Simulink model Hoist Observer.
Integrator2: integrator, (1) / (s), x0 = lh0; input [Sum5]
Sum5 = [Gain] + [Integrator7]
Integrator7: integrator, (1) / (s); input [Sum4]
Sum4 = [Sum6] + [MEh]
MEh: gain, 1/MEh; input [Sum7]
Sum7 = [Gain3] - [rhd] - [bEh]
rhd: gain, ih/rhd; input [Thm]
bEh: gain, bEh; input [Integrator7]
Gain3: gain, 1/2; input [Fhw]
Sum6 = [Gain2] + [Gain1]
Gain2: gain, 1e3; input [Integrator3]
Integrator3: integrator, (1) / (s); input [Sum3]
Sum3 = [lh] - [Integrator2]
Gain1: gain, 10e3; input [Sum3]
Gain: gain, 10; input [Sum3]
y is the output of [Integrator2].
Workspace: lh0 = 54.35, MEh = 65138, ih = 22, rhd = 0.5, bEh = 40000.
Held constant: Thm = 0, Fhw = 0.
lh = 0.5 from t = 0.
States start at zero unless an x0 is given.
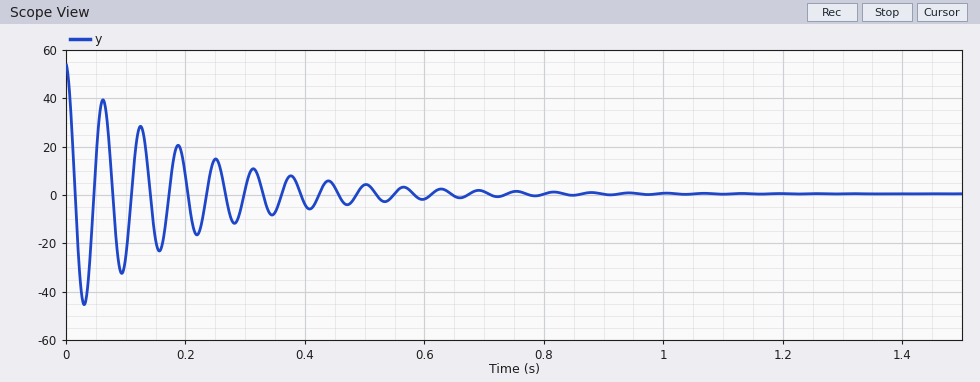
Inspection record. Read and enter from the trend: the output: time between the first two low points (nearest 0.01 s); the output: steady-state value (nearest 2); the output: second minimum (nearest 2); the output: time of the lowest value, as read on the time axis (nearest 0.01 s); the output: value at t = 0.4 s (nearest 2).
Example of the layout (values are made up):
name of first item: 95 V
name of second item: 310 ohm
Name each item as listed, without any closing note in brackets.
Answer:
the output: time between the first two low points: 0.06 s
the output: steady-state value: 0
the output: second minimum: -32
the output: time of the lowest value, as read on the time axis: 0.03 s
the output: value at t = 0.4 s: -4
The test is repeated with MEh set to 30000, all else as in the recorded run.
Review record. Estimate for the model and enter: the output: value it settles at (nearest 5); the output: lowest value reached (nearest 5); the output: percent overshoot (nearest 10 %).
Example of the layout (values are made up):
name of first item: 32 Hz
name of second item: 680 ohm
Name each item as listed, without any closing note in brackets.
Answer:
the output: value it settles at: 0
the output: lowest value reached: -45
the output: percent overshoot: 80 %
